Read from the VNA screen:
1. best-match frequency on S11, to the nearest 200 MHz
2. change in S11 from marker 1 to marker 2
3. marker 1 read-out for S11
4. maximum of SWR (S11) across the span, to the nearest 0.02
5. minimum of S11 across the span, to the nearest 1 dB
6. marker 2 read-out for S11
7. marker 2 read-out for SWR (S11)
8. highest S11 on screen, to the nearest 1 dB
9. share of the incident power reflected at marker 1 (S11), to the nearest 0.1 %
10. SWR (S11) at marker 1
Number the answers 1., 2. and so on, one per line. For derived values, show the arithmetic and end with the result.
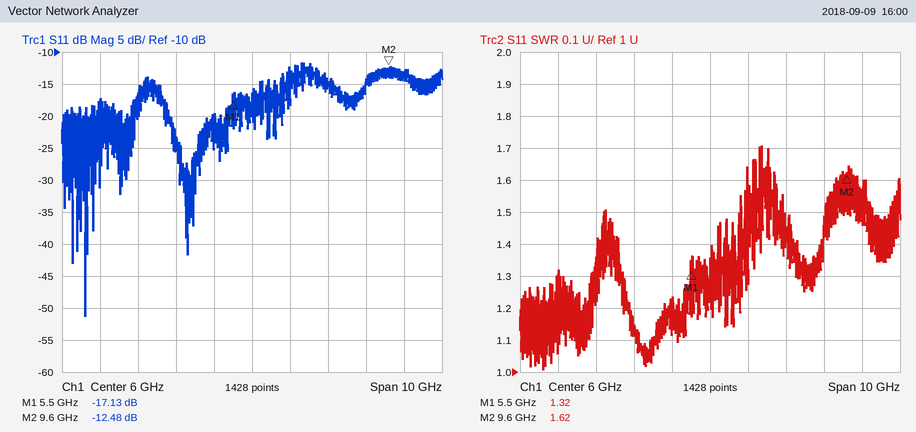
1. 1.6 GHz
2. -12.48 − (-17.13) = 4.65 dB
3. -17.13 dB
4. 1.70
5. -51 dB
6. -12.48 dB
7. 1.62
8. -12 dB
9. 10^(-17.13/10) ≈ 1.9 %
10. 1.32
